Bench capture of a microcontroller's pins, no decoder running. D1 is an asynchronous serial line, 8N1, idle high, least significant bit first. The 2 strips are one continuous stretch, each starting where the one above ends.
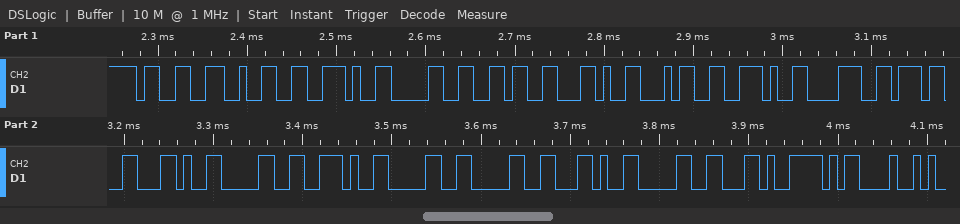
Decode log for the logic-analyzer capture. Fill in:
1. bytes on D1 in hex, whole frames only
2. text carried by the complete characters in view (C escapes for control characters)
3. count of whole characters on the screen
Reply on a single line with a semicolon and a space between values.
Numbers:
33 32 2E 30 36 2C 34 2E 38 37 2C 30 2E 30 30 2C 30 2C 0D; "32.06,4.87,0.00,0,\r"; 19
